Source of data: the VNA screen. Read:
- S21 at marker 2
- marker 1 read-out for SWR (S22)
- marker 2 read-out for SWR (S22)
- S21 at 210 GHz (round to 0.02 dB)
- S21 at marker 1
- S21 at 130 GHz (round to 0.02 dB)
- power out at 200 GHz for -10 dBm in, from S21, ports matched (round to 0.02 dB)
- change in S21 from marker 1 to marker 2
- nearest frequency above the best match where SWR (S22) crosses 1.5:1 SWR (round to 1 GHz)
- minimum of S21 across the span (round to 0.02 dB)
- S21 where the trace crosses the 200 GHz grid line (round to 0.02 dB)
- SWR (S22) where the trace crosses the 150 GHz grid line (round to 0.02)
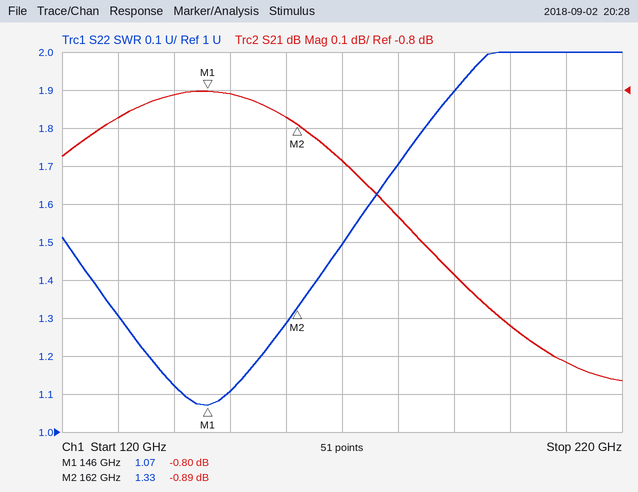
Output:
-0.89 dB
1.07
1.33
-1.52 dB
-0.80 dB
-0.88 dB
-11.42 dBm
-0.09 dB
170 GHz
-1.56 dB
-1.42 dB
1.10
